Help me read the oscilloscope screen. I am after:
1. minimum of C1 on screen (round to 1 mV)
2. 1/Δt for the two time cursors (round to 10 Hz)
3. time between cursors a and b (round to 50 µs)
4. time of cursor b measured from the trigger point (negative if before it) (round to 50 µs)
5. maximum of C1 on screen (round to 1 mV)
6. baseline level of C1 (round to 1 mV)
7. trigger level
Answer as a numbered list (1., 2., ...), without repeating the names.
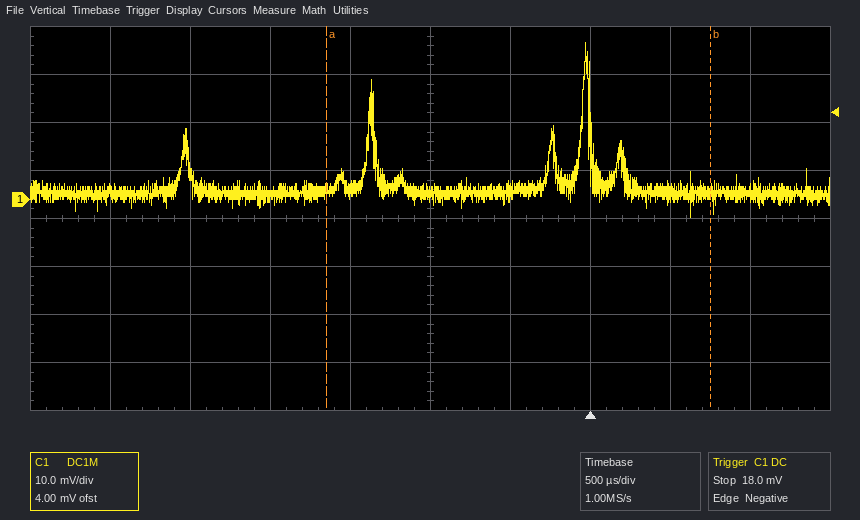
1. -4 mV
2. 420 Hz
3. 2.40 ms
4. +750 µs
5. 33 mV
6. 1 mV
7. 18.0 mV
